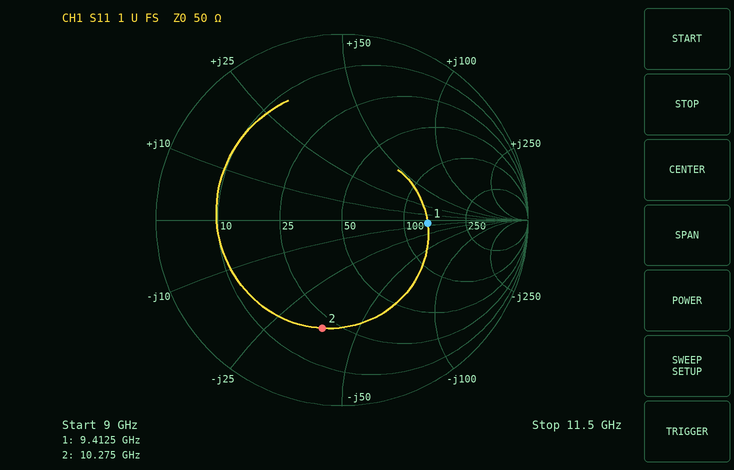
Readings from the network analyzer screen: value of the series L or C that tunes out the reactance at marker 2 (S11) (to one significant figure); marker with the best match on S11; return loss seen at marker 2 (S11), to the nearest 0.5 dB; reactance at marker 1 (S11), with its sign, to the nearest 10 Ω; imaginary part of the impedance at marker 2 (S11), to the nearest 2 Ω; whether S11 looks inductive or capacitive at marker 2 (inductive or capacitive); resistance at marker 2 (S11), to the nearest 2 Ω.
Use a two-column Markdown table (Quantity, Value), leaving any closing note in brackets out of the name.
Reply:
| Quantity | Value |
|---|---|
| value of the series L or C that tunes out the reactance at marker 2 (S11) | 600 pH |
| marker with the best match on S11 | marker 1 |
| return loss seen at marker 2 (S11), to the nearest 0.5 dB | 4.5 dB |
| reactance at marker 1 (S11), with its sign, to the nearest 10 Ω | -10 Ω |
| imaginary part of the impedance at marker 2 (S11), to the nearest 2 Ω | -38 Ω |
| whether S11 looks inductive or capacitive at marker 2 | capacitive |
| resistance at marker 2 (S11), to the nearest 2 Ω | 20 Ω |
